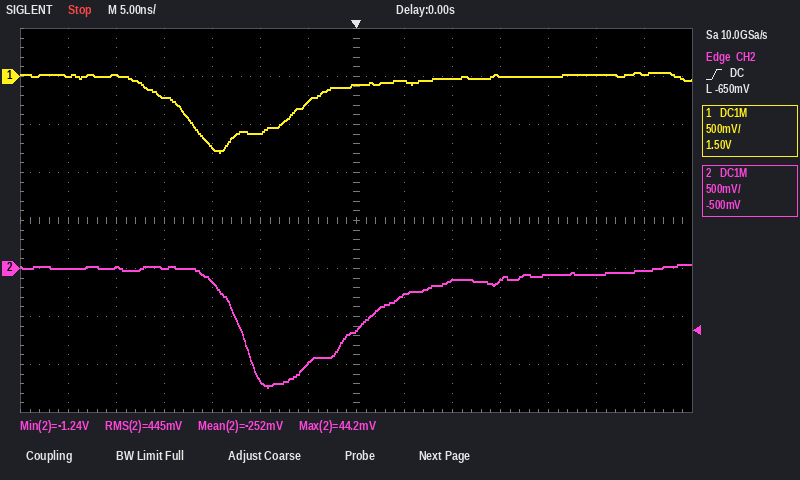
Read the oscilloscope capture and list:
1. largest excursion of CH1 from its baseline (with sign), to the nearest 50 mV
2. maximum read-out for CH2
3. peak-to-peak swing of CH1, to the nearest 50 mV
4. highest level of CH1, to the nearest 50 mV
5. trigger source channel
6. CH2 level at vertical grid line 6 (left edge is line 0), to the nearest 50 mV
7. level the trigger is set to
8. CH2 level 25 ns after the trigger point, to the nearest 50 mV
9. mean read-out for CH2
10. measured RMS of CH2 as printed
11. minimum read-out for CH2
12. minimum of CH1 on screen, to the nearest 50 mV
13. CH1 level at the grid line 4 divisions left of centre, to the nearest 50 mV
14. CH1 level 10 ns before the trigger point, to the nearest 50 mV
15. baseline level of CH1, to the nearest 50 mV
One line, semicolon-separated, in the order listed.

-800 mV; 44.2 mV; 850 mV; 50 mV; CH2; -1.00 V; -650 mV; -50 mV; -252 mV; 445 mV; -1.24 V; -800 mV; -200 mV; -600 mV; 0 mV
